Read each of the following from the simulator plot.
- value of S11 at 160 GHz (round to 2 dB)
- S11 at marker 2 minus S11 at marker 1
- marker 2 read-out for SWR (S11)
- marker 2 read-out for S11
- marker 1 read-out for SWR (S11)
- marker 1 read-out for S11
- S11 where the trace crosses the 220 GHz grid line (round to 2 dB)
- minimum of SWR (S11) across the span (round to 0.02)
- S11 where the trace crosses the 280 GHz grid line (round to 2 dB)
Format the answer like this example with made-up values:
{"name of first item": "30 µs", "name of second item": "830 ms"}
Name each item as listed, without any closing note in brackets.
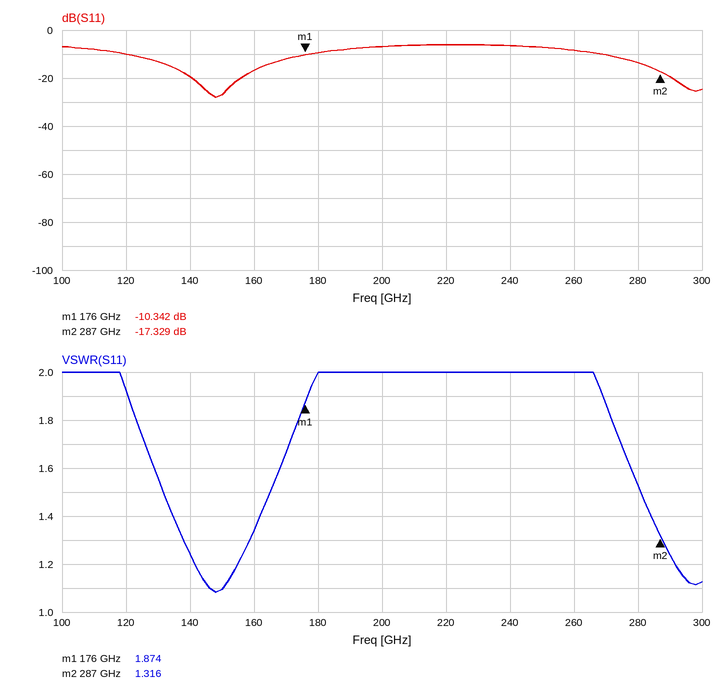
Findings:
{"value of S11 at 160 GHz": "-16 dB", "S11 at marker 2 minus S11 at marker 1": "-6.987 dB", "marker 2 read-out for SWR": "1.316", "marker 2 read-out for S11": "-17.329 dB", "marker 1 read-out for SWR": "1.874", "marker 1 read-out for S11": "-10.342 dB", "S11 where the trace crosses the 220 GHz grid line": "-6 dB", "minimum of SWR (S11) across the span": "1.08", "S11 where the trace crosses the 280 GHz grid line": "-14 dB"}
